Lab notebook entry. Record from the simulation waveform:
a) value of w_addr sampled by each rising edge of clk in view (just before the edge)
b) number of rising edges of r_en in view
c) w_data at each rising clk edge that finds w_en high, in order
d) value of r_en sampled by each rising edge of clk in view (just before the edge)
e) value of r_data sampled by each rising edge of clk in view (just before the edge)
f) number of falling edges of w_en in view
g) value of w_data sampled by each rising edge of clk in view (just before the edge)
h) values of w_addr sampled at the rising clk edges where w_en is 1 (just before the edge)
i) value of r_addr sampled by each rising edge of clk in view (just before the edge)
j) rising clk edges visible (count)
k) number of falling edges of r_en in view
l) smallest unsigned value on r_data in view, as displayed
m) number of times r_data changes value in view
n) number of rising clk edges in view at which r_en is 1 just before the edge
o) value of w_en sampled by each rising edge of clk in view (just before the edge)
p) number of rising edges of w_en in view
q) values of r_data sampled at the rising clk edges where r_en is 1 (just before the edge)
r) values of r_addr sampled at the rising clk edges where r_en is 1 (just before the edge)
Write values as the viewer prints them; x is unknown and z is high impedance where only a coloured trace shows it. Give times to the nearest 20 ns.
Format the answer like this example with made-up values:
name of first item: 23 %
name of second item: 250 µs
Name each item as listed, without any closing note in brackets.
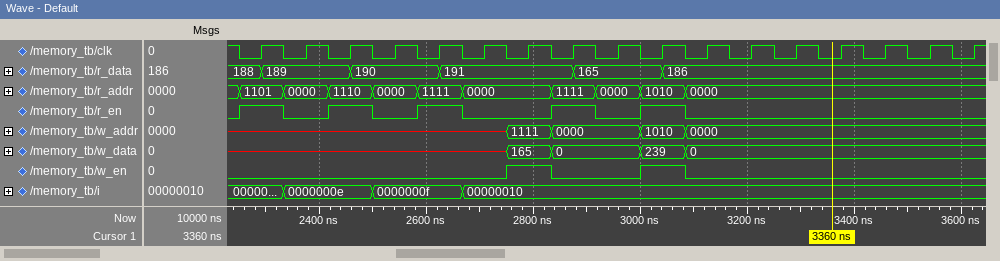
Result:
value of w_addr sampled by each rising edge of clk in view: x, x, x, x, x, x, 1111, 0000, 0000, 1010, 0000, 0000, 0000, 0000, 0000, 0000, 0000
number of rising edges of r_en in view: 5
w_data at each rising clk edge that finds w_en high, in order: 165, 239
value of r_en sampled by each rising edge of clk in view: 1 0 1 0 1 0 0 1 0 1 0 0 0 0 0 0 0
value of r_data sampled by each rising edge of clk in view: 188, 189, 189, 190, 190, 191, 191, 191, 165, 165, 186, 186, 186, 186, 186, 186, 186
number of falling edges of w_en in view: 2
value of w_data sampled by each rising edge of clk in view: x, x, x, x, x, x, 165, 0, 0, 239, 0, 0, 0, 0, 0, 0, 0
values of w_addr sampled at the rising clk edges where w_en is 1: 1111, 1010
value of r_addr sampled by each rising edge of clk in view: 1101, 0000, 1110, 0000, 1111, 0000, 0000, 1111, 0000, 1010, 0000, 0000, 0000, 0000, 0000, 0000, 0000
rising clk edges visible: 17
number of falling edges of r_en in view: 5
smallest unsigned value on r_data in view, as displayed: 165
number of times r_data changes value in view: 5
number of rising clk edges in view at which r_en is 1 just before the edge: 5
value of w_en sampled by each rising edge of clk in view: 0 0 0 0 0 0 1 0 0 1 0 0 0 0 0 0 0
number of rising edges of w_en in view: 2
values of r_data sampled at the rising clk edges where r_en is 1: 188, 189, 190, 191, 165
values of r_addr sampled at the rising clk edges where r_en is 1: 1101, 1110, 1111, 1111, 1010
